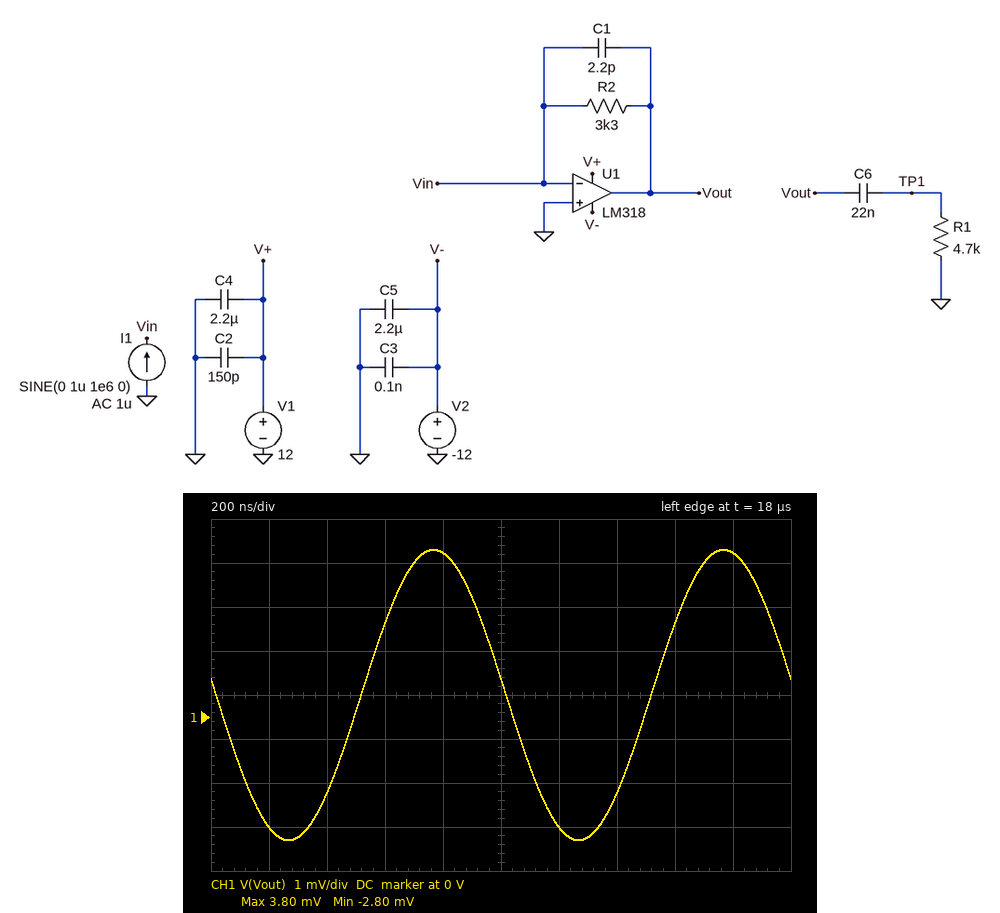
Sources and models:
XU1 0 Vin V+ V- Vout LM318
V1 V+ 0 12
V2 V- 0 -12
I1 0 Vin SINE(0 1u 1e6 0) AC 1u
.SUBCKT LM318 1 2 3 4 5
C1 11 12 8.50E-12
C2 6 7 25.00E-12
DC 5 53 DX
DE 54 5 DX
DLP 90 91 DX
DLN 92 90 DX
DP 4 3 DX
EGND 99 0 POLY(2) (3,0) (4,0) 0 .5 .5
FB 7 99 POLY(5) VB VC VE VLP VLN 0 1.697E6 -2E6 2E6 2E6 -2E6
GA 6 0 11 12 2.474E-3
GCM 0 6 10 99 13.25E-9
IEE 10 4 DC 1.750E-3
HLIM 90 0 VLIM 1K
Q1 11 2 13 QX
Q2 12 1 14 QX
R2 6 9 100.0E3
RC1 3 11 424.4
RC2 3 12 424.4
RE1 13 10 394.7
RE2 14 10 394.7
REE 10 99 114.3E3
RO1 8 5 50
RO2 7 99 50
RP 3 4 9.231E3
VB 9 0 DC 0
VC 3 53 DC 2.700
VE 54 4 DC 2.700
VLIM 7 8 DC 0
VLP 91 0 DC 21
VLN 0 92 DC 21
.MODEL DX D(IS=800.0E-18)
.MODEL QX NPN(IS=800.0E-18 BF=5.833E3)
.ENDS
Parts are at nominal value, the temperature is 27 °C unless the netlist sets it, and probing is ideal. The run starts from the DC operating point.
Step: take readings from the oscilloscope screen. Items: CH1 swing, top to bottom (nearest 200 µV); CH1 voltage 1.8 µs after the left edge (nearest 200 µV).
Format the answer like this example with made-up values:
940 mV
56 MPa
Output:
6.6 mV
3.8 mV
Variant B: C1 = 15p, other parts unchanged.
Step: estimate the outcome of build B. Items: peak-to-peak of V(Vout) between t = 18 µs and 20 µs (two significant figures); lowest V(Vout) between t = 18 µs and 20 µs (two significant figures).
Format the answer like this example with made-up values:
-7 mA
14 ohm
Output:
6.3 mV
-2.7 mV
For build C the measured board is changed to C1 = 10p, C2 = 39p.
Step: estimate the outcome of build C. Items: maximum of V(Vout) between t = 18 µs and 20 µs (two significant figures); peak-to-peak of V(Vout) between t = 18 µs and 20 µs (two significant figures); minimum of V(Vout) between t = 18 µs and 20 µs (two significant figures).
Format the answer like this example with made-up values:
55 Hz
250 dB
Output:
3.7 mV
6.5 mV
-2.7 mV
